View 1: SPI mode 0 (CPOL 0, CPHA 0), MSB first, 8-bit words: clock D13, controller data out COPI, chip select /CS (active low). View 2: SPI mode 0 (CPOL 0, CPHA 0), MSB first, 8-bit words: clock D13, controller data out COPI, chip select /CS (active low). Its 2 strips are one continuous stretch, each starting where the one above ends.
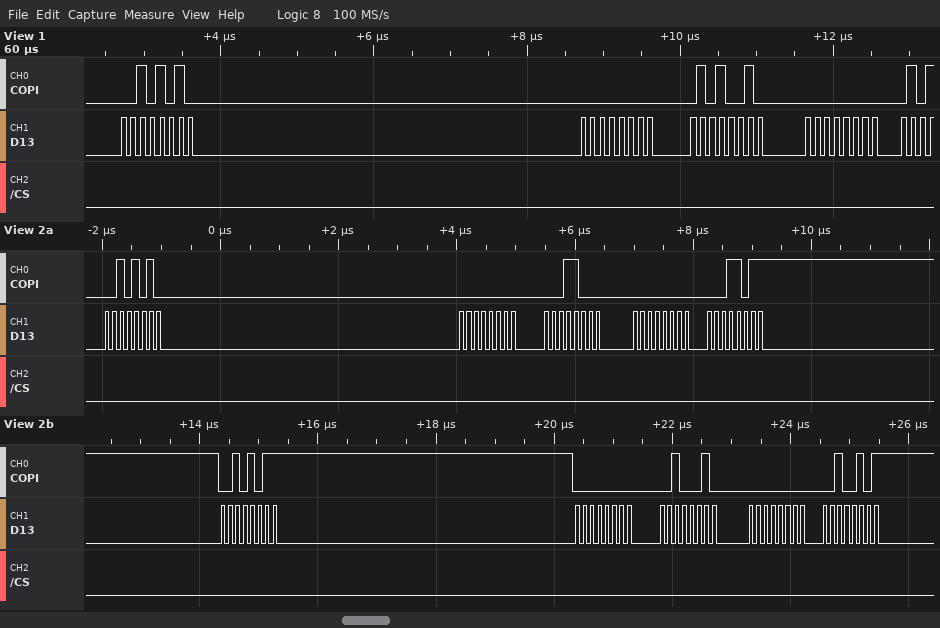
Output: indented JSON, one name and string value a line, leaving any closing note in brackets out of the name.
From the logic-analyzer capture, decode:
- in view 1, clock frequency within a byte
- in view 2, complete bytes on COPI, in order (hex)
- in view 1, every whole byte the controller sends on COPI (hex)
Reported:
{
  "in view 1, clock frequency within a byte": "8 MHz",
  "in view 2, complete bytes on COPI, in order": "2A 00 18 00 1B 2B 00 22 00 25",
  "in view 1, every whole byte the controller sends on COPI": "2A 00 52 00"
}
